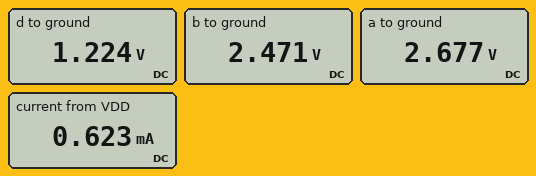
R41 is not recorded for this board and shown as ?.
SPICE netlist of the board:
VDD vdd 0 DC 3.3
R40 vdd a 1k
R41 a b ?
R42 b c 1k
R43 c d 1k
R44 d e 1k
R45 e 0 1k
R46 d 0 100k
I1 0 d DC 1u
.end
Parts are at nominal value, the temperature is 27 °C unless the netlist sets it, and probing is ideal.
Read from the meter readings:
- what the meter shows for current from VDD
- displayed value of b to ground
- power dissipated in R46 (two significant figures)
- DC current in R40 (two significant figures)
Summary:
0.623 mA
2.471 V
15 µW
620 µA
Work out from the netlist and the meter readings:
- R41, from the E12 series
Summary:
330 Ω
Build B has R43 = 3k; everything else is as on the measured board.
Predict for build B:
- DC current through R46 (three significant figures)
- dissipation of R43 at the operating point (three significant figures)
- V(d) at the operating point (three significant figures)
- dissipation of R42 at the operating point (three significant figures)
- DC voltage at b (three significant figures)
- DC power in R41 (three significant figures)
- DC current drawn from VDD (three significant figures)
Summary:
8.89 µA
614 µW
889 mV
205 µW
2.70 V
67.5 µW
452 µA
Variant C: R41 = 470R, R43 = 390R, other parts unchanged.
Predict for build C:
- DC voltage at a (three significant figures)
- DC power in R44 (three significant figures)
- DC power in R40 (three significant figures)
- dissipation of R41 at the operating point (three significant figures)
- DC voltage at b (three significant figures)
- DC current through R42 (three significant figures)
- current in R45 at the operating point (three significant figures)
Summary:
2.62 V
451 µW
468 µW
220 µW
2.29 V
684 µA
672 µA
